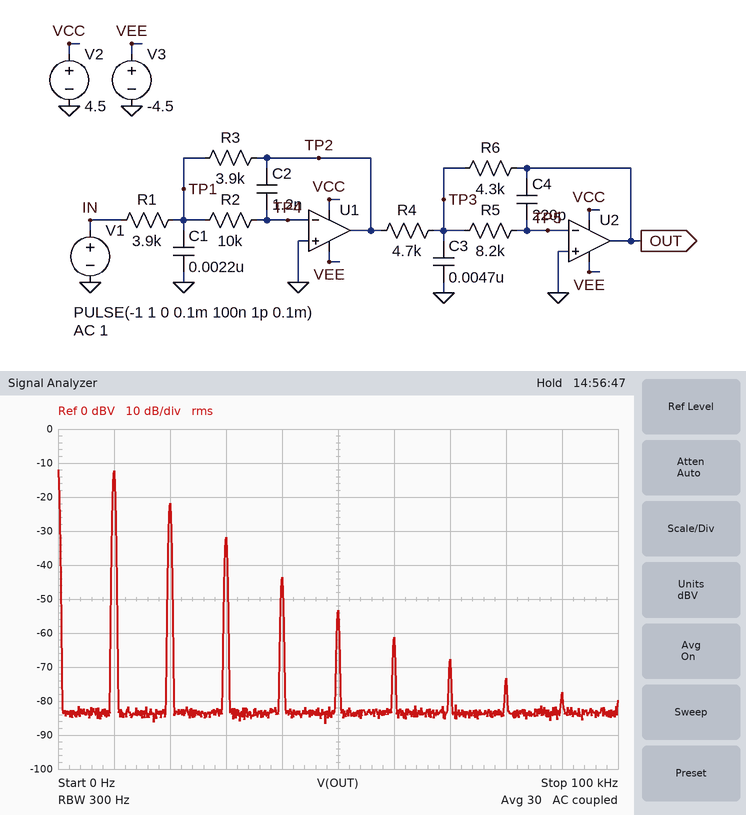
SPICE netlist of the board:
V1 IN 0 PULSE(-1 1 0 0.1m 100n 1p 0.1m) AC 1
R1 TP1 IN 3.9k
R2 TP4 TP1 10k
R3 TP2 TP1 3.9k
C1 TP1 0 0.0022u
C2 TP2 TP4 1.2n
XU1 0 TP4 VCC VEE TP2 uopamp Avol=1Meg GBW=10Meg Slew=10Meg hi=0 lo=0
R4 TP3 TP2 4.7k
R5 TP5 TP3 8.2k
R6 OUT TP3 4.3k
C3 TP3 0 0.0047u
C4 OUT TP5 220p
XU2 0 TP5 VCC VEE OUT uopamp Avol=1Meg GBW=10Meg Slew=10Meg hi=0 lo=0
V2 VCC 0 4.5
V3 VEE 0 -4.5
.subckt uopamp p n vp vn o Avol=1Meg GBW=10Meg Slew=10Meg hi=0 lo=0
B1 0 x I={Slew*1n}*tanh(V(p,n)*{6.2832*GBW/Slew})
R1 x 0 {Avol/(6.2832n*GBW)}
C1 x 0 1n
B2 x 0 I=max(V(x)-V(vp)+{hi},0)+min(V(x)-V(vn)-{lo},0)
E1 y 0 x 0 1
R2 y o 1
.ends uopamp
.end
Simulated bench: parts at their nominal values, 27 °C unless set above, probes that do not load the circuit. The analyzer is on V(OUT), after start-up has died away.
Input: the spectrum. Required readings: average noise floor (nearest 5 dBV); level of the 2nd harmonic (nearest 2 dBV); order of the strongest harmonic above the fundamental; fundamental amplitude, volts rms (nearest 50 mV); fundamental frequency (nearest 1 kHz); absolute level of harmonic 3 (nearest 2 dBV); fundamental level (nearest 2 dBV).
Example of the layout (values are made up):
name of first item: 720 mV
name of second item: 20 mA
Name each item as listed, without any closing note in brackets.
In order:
average noise floor: -85 dBV
level of the 2nd harmonic: -22 dBV
order of the strongest harmonic above the fundamental: 2
fundamental amplitude, volts rms: 250 mV
fundamental frequency: 10 kHz
absolute level of harmonic 3: -32 dBV
fundamental level: -12 dBV
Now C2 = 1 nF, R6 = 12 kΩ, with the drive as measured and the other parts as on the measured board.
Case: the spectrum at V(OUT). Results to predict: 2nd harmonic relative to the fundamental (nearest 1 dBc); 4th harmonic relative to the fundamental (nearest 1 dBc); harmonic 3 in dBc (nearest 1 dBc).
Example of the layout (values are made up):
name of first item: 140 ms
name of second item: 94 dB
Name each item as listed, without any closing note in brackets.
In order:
2nd harmonic relative to the fundamental: -15 dBc
4th harmonic relative to the fundamental: -42 dBc
harmonic 3 in dBc: -31 dBc
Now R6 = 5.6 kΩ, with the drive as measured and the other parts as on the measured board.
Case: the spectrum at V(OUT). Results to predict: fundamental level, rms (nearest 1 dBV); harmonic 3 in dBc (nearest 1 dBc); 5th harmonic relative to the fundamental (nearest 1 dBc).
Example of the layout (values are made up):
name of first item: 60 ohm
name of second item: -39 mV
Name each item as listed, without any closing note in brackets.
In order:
fundamental level, rms: -10 dBV
harmonic 3 in dBc: -22 dBc
5th harmonic relative to the fundamental: -44 dBc
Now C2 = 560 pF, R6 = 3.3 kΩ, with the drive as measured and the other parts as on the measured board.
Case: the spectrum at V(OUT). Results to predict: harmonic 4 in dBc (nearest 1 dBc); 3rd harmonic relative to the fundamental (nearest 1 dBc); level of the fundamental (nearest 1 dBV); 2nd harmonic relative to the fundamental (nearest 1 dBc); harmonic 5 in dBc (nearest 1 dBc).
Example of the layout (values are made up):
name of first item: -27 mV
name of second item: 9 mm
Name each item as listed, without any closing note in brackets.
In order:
harmonic 4 in dBc: -25 dBc
3rd harmonic relative to the fundamental: -14 dBc
level of the fundamental: -11 dBV
2nd harmonic relative to the fundamental: -7 dBc
harmonic 5 in dBc: -35 dBc
